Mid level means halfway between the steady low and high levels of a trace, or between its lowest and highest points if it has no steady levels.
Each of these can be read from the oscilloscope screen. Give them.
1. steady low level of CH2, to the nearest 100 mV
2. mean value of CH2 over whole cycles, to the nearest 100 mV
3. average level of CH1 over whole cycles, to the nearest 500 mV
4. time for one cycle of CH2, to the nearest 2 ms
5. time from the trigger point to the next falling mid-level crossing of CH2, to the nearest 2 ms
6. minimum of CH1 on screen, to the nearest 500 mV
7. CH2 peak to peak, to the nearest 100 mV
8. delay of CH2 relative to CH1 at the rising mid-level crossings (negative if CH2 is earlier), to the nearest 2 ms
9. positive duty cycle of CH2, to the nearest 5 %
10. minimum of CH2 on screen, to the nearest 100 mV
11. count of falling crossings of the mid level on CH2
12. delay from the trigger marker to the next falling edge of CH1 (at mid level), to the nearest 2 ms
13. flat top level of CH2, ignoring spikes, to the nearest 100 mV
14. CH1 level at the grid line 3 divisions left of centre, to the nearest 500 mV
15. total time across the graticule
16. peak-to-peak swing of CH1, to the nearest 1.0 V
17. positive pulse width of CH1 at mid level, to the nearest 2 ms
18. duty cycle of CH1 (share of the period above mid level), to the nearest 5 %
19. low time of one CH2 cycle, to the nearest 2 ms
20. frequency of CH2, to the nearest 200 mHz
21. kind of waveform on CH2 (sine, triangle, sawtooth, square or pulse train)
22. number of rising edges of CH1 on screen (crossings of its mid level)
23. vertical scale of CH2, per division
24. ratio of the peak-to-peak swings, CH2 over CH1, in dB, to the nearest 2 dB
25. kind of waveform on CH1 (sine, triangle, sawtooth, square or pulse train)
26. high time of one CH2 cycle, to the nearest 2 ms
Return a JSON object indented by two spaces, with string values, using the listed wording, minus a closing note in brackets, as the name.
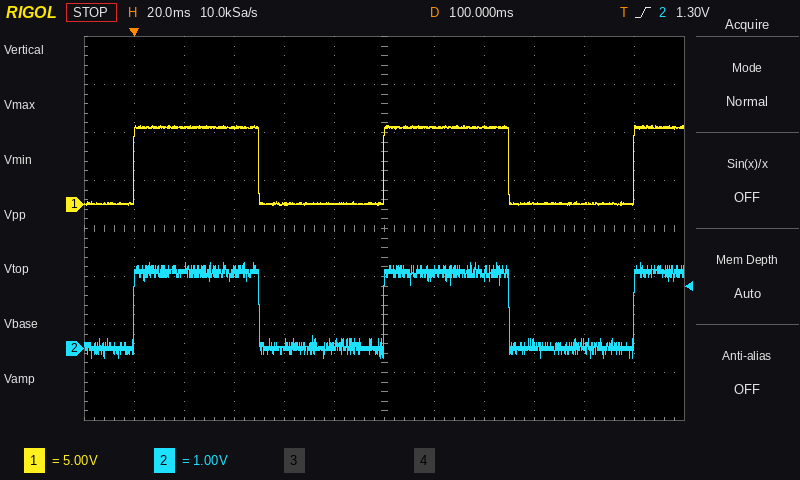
{
  "steady low level of CH2, to the nearest 100 mV": "0.0 V",
  "mean value of CH2 over whole cycles, to the nearest 100 mV": "800 mV",
  "average level of CH1 over whole cycles, to the nearest 500 mV": "4.0 V",
  "time for one cycle of CH2, to the nearest 2 ms": "100 ms",
  "time from the trigger point to the next falling mid-level crossing of CH2, to the nearest 2 ms": "50 ms",
  "minimum of CH1 on screen, to the nearest 500 mV": "0.0 V",
  "CH2 peak to peak, to the nearest 100 mV": "2.0 V",
  "delay of CH2 relative to CH1 at the rising mid-level crossings (negative if CH2 is earlier), to the nearest 2 ms": "0 ms",
  "positive duty cycle of CH2, to the nearest 5 %": "50 %",
  "minimum of CH2 on screen, to the nearest 100 mV": "-200 mV",
  "count of falling crossings of the mid level on CH2": "2",
  "delay from the trigger marker to the next falling edge of CH1 (at mid level), to the nearest 2 ms": "50 ms",
  "flat top level of CH2, ignoring spikes, to the nearest 100 mV": "1.6 V",
  "CH1 level at the grid line 3 divisions left of centre, to the nearest 500 mV": "8.0 V",
  "total time across the graticule": "240 ms",
  "peak-to-peak swing of CH1, to the nearest 1.0 V": "8.0 V",
  "positive pulse width of CH1 at mid level, to the nearest 2 ms": "50 ms",
  "duty cycle of CH1 (share of the period above mid level), to the nearest 5 %": "50 %",
  "low time of one CH2 cycle, to the nearest 2 ms": "50 ms",
  "frequency of CH2, to the nearest 200 mHz": "10.0 Hz",
  "kind of waveform on CH2": "square",
  "number of rising edges of CH1 on screen": "3",
  "vertical scale of CH2, per division": "1 V",
  "ratio of the peak-to-peak swings, CH2 over CH1, in dB, to the nearest 2 dB": "-12 dB",
  "kind of waveform on CH1": "square",
  "high time of one CH2 cycle, to the nearest 2 ms": "50 ms"
}
